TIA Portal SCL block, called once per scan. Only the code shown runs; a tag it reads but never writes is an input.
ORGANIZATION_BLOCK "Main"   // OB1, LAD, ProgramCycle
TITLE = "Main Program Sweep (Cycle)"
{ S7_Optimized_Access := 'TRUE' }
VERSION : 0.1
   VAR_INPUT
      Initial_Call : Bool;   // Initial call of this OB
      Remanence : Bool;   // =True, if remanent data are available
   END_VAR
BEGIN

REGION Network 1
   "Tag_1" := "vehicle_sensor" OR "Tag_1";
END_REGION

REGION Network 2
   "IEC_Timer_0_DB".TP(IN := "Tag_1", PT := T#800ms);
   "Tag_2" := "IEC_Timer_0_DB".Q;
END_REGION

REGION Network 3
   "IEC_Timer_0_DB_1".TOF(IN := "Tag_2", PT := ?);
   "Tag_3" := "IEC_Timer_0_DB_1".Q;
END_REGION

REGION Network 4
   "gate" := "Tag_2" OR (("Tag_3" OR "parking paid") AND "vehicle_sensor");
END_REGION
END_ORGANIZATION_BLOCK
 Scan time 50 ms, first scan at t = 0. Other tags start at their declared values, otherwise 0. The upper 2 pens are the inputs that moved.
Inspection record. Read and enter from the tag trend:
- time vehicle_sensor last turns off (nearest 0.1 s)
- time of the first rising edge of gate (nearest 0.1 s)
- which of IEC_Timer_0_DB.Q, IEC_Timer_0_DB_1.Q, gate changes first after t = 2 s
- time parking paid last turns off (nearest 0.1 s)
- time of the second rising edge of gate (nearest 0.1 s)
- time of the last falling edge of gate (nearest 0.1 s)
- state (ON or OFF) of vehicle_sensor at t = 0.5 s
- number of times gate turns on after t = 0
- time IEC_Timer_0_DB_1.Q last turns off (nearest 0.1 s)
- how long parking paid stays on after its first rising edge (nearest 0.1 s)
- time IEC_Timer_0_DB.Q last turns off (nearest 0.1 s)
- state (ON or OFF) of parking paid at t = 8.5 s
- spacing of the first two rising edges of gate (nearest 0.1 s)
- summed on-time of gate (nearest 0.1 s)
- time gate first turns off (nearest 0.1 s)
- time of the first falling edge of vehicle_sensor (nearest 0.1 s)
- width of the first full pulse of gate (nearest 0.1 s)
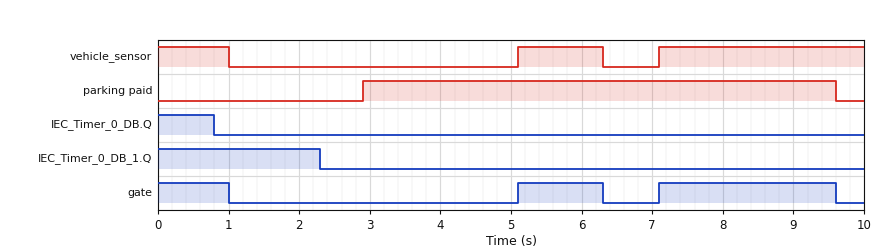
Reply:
6.3 s
5.1 s
IEC_Timer_0_DB_1.Q
9.6 s
7.1 s
9.6 s
ON
2
2.3 s
6.7 s
0.8 s
ON
2.0 s
4.7 s
1.0 s
1.0 s
1.2 s
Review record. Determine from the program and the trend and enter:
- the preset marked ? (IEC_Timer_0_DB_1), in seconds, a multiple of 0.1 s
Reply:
1.5 s
